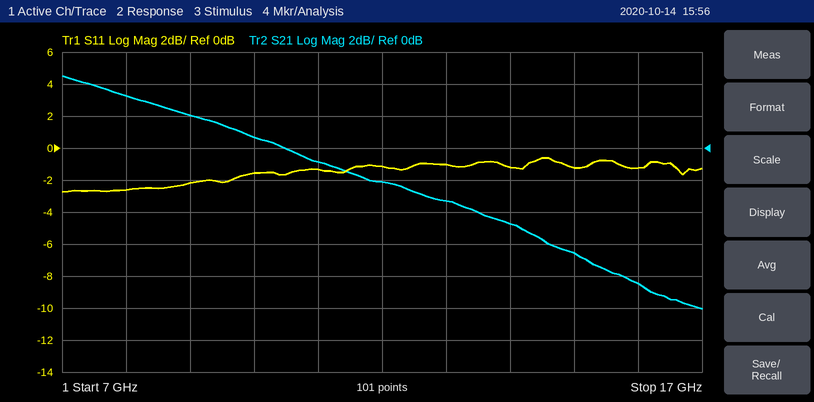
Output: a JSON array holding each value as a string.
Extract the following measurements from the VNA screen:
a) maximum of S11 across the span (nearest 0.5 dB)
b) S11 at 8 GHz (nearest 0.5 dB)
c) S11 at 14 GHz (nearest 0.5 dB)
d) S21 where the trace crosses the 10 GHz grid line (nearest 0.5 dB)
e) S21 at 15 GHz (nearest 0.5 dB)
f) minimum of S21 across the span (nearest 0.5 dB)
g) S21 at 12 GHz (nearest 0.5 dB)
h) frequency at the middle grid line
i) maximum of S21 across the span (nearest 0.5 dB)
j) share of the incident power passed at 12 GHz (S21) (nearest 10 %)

["-0.5 dB", "-2.5 dB", "-1.0 dB", "0.5 dB", "-6.5 dB", "-10.0 dB", "-2.0 dB", "12 GHz", "4.5 dB", "60 %"]
